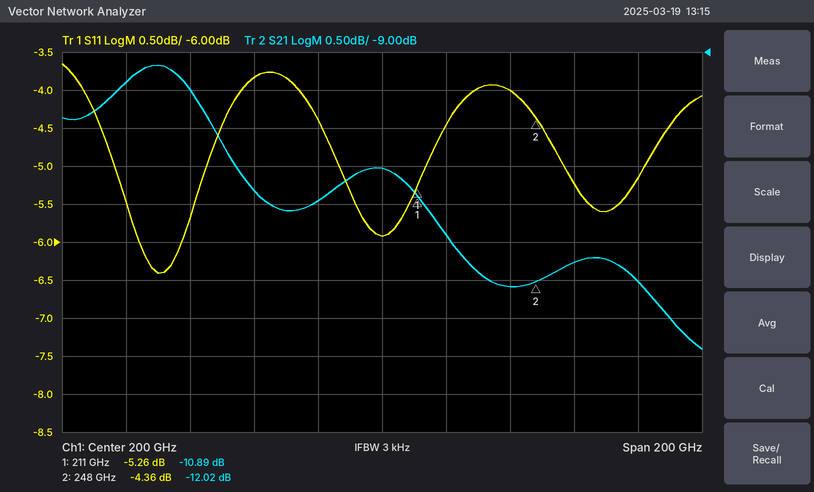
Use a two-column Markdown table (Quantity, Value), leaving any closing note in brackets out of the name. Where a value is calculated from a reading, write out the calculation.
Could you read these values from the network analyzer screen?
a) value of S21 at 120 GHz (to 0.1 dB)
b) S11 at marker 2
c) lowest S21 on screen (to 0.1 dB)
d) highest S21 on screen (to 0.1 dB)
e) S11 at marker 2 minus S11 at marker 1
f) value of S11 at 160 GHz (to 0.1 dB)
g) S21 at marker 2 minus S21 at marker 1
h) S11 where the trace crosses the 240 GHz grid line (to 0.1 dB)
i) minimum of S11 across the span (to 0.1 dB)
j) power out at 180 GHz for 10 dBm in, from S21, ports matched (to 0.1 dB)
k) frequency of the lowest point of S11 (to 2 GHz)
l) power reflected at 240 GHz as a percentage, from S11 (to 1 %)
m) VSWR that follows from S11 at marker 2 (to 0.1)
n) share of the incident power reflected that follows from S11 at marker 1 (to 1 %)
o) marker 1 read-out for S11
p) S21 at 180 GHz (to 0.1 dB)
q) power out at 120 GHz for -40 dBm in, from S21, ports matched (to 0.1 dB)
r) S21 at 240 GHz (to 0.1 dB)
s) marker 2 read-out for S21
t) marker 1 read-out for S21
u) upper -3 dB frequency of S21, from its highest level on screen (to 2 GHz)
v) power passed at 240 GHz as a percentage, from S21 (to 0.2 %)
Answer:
| Quantity | Value |
|---|---|
| value of S21 at 120 GHz | -9.4 dB |
| S11 at marker 2 | -4.36 dB |
| lowest S21 on screen | -12.9 dB |
| highest S21 on screen | -9.2 dB |
| S11 at marker 2 minus S11 at marker 1 | -4.36 − (-5.26) = 0.90 dB |
| value of S11 at 160 GHz | -3.8 dB |
| S21 at marker 2 minus S21 at marker 1 | -12.02 − (-10.89) = -1.13 dB |
| S11 where the trace crosses the 240 GHz grid line | -4.0 dB |
| minimum of S11 across the span | -6.4 dB |
| power out at 180 GHz for 10 dBm in, from S21, ports matched | 10 dBm + (-11.0 dB) = -1.0 dBm |
| frequency of the lowest point of S11 | 130 GHz |
| power reflected at 240 GHz as a percentage, from S11 | 10^(-4/10) ≈ 40 % |
| VSWR that follows from S11 at marker 2 | (1 + 0.6053)/(1 − 0.6053) ≈ 4.1 |
| share of the incident power reflected that follows from S11 at marker 1 | 10^(-5.26/10) ≈ 30 % |
| marker 1 read-out for S11 | -5.26 dB |
| S21 at 180 GHz | -11.0 dB |
| power out at 120 GHz for -40 dBm in, from S21, ports matched | -40 dBm + (-9.4 dB) = -49.4 dBm |
| S21 at 240 GHz | -12.1 dB |
| marker 2 read-out for S21 | -12.02 dB |
| marker 1 read-out for S21 | -10.89 dB |
| upper -3 dB frequency of S21, from its highest level on screen | 284 GHz |
| power passed at 240 GHz as a percentage, from S21 | 10^(-12.1/10) ≈ 6.2 % |
